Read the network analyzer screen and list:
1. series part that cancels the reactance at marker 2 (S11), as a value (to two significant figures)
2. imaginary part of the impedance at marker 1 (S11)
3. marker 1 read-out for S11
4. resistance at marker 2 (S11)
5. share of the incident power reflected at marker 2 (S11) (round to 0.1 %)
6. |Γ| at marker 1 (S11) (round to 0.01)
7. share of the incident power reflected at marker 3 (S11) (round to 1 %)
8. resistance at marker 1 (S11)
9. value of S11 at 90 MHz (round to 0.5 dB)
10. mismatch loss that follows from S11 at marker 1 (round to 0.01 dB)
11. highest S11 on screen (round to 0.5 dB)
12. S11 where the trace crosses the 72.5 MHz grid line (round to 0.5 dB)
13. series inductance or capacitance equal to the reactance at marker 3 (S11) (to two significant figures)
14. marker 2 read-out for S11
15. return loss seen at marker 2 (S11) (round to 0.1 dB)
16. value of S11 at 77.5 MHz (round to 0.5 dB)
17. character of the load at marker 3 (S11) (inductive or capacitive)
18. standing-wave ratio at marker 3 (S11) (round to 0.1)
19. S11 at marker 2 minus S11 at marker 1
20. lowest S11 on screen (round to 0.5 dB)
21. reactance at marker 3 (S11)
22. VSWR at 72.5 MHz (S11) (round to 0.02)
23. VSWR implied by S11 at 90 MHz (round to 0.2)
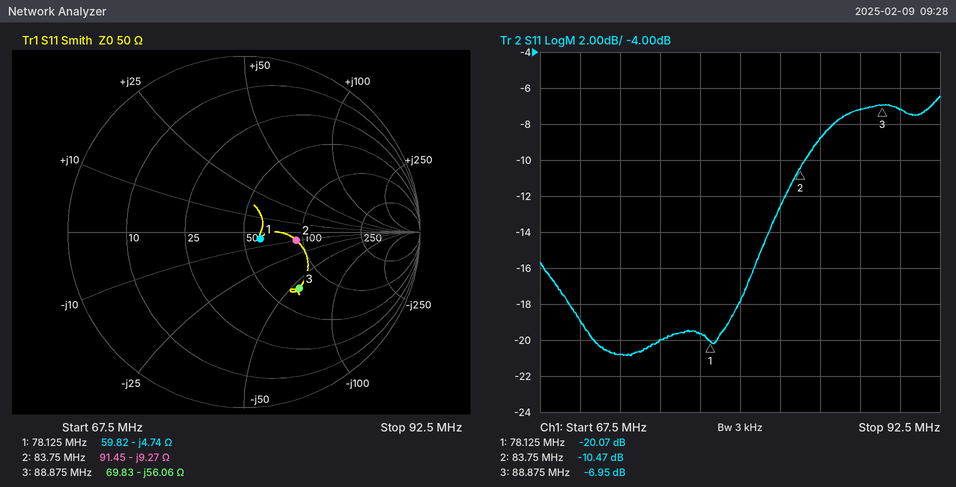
18 nH
-4.74 Ω
-20.07 dB
91.45 Ω
9.0 %
0.10
20 %
59.82 Ω
-7.0 dB
0.04 dB
-6.5 dB
-21.0 dB
32 pF
-10.47 dB
10.5 dB
-19.5 dB
capacitive
2.6
9.60 dB
-21.0 dB
-56.06 Ω
1.20
2.6
